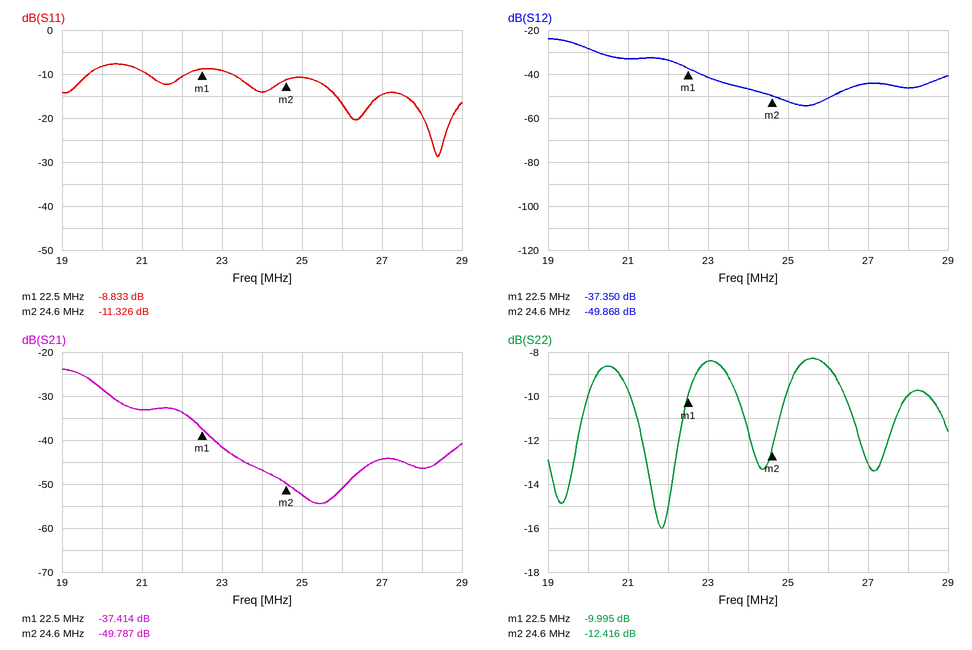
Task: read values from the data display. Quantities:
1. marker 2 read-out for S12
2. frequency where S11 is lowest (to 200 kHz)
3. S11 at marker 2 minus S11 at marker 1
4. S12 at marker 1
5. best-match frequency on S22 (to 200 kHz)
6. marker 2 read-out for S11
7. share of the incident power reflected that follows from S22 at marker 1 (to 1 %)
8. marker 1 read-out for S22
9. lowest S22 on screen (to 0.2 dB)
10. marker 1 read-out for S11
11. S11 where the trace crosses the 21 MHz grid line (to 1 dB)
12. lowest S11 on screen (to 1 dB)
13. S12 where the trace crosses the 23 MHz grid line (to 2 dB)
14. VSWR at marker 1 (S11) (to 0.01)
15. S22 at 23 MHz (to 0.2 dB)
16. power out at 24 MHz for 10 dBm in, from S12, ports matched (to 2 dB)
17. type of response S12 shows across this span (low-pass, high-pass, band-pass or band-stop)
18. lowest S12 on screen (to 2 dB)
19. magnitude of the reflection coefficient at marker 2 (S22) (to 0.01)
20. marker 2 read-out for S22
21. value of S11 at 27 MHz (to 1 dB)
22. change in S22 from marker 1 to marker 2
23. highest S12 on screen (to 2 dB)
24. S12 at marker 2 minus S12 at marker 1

-49.868 dB
28.4 MHz
-2.493 dB
-37.350 dB
21.8 MHz
-11.326 dB
10 %
-9.995 dB
-16.0 dB
-8.833 dB
-9 dB
-29 dB
-42 dB
2.13
-8.4 dB
-36 dBm
low-pass
-54 dB
0.24
-12.416 dB
-15 dB
-2.421 dB
-24 dB
-12.518 dB
